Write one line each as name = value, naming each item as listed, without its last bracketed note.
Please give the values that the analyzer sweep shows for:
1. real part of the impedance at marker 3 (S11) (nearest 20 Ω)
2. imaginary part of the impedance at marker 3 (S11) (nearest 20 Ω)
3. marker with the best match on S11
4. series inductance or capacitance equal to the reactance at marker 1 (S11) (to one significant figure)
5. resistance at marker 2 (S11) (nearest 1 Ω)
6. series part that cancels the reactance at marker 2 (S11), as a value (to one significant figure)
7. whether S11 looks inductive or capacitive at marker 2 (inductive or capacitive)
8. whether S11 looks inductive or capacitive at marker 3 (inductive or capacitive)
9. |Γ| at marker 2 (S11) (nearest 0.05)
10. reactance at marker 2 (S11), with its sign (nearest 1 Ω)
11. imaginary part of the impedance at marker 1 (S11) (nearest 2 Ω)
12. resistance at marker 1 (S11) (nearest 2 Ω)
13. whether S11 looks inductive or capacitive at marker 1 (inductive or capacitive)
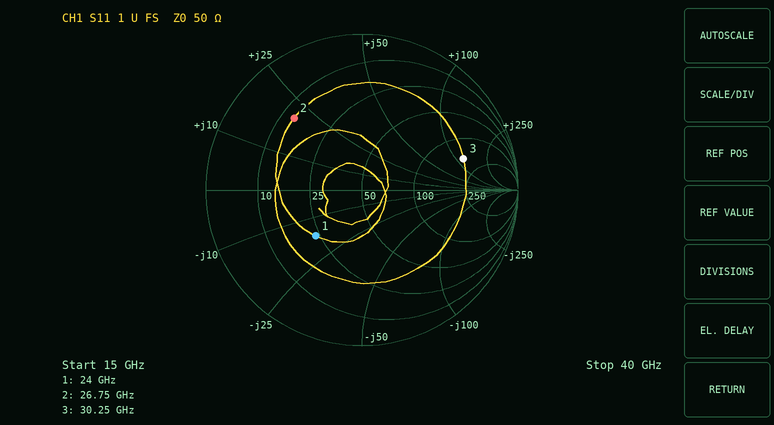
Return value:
real part of the impedance at marker 3 (S11) = 160 Ω
imaginary part of the impedance at marker 3 (S11) = +120 Ω
marker with the best match on S11 = marker 1
series inductance or capacitance equal to the reactance at marker 1 (S11) = 400 fF
resistance at marker 2 (S11) = 13 Ω
series part that cancels the reactance at marker 2 (S11), as a value = 300 fF
whether S11 looks inductive or capacitive at marker 2 = inductive
whether S11 looks inductive or capacitive at marker 3 = inductive
|Γ| at marker 2 (S11) = 0.65
reactance at marker 2 (S11), with its sign = +20 Ω
imaginary part of the impedance at marker 1 (S11) = -16 Ω
resistance at marker 1 (S11) = 24 Ω
whether S11 looks inductive or capacitive at marker 1 = capacitive
